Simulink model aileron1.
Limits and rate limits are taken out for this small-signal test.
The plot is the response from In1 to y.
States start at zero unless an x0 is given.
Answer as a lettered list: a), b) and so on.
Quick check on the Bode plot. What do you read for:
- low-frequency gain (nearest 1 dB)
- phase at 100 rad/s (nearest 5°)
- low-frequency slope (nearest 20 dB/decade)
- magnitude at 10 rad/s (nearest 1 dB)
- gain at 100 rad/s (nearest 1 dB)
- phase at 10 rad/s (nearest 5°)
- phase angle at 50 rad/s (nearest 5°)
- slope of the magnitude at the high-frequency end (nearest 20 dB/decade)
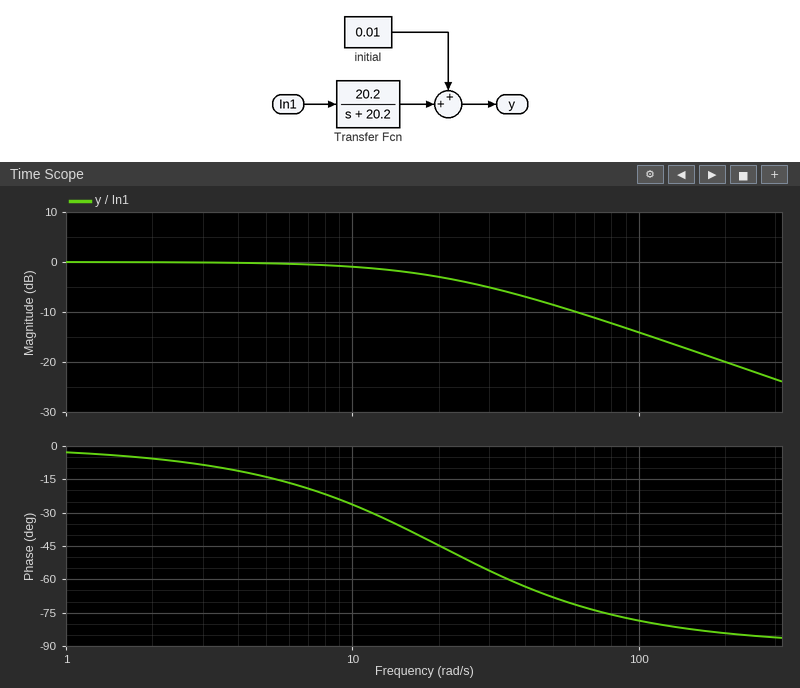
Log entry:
a) 0 dB
b) -80°
c) 0 dB/decade
d) -1 dB
e) -14 dB
f) -25°
g) -70°
h) -20 dB/decade
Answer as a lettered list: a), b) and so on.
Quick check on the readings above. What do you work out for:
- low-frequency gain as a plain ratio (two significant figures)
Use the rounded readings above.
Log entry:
a) 1.0
